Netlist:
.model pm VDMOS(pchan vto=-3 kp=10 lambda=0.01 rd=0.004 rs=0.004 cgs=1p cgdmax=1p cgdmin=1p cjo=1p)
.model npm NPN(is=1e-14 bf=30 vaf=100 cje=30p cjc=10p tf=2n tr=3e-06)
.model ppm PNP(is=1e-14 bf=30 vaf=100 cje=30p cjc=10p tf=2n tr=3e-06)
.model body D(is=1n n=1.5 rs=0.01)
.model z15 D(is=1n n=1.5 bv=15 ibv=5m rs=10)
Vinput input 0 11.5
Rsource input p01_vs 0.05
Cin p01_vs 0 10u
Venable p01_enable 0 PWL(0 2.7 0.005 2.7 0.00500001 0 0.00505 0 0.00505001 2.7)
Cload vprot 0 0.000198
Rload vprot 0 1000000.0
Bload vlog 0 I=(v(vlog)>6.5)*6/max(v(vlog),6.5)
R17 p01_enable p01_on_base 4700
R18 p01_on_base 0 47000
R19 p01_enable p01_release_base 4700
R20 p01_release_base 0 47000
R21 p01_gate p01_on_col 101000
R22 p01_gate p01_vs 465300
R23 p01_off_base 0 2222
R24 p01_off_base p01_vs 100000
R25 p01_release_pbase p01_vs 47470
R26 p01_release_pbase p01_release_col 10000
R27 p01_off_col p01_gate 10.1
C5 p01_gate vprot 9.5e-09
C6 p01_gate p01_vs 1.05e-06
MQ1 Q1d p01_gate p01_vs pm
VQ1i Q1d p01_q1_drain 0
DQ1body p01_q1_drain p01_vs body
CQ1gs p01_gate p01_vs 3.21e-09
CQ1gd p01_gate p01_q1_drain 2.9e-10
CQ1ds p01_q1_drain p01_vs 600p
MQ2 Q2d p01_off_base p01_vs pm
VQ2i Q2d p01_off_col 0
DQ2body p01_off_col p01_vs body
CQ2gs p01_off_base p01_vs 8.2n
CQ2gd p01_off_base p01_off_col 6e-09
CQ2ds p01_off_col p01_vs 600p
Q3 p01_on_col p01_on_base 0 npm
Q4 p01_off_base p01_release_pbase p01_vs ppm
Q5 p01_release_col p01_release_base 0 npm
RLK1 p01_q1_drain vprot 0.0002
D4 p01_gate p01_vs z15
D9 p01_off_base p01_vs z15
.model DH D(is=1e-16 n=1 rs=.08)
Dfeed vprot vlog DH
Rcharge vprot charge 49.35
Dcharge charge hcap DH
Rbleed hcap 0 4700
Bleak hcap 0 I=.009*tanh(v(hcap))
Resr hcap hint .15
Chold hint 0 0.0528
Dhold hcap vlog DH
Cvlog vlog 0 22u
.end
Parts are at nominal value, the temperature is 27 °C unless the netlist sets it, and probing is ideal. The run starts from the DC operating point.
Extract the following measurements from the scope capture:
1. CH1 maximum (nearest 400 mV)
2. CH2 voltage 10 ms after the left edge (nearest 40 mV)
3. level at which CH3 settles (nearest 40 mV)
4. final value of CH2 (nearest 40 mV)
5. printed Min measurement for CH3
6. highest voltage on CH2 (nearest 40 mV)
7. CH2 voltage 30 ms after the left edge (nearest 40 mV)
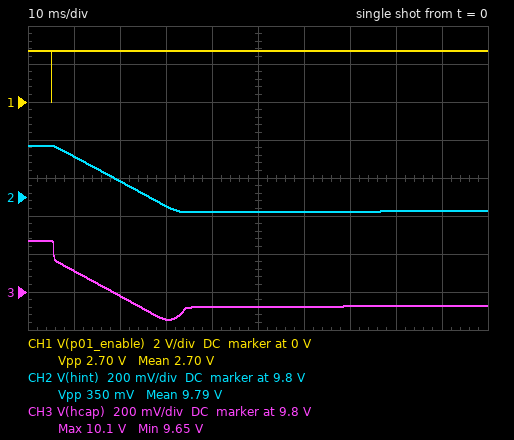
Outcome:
2.8 V
10.00 V
9.72 V
9.72 V
9.65 V
10.08 V
9.76 V
